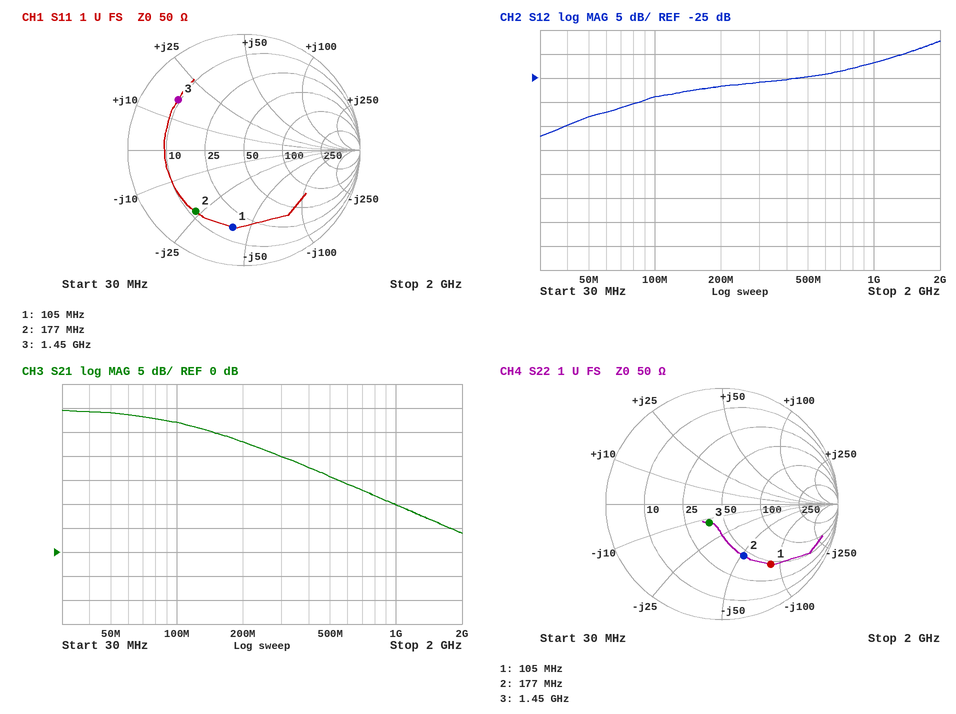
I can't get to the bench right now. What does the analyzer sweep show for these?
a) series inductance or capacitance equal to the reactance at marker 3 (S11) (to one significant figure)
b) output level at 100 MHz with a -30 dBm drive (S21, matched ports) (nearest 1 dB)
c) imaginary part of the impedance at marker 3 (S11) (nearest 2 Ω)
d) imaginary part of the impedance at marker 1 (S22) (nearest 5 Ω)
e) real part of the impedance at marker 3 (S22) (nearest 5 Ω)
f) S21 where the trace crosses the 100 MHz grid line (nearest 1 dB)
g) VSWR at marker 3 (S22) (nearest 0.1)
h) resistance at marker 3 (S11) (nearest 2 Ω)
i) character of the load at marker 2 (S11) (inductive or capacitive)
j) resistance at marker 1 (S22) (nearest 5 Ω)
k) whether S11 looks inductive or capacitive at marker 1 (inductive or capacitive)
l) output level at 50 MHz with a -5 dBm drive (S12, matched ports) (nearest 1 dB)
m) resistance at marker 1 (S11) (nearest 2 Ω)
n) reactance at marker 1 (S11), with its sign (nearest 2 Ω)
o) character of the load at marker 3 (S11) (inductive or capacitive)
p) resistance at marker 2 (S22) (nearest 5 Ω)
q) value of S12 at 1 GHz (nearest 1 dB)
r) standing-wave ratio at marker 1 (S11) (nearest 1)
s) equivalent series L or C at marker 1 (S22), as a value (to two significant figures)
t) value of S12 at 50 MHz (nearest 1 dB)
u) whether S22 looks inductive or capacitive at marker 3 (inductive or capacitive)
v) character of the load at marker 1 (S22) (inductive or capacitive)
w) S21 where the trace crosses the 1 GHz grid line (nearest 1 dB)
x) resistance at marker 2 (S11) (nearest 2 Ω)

2 nH
-3 dBm
+16 Ω
-85 Ω
40 Ω
27 dB
1.5
10 Ω
capacitive
45 Ω
capacitive
-38 dBm
16 Ω
-40 Ω
inductive
45 Ω
-22 dB
5
18 pF
-33 dB
capacitive
capacitive
10 dB
12 Ω
